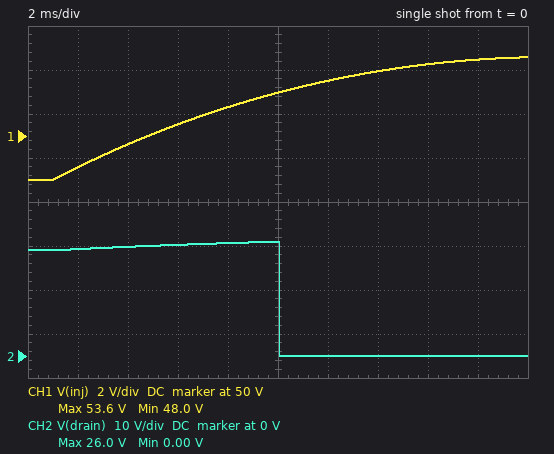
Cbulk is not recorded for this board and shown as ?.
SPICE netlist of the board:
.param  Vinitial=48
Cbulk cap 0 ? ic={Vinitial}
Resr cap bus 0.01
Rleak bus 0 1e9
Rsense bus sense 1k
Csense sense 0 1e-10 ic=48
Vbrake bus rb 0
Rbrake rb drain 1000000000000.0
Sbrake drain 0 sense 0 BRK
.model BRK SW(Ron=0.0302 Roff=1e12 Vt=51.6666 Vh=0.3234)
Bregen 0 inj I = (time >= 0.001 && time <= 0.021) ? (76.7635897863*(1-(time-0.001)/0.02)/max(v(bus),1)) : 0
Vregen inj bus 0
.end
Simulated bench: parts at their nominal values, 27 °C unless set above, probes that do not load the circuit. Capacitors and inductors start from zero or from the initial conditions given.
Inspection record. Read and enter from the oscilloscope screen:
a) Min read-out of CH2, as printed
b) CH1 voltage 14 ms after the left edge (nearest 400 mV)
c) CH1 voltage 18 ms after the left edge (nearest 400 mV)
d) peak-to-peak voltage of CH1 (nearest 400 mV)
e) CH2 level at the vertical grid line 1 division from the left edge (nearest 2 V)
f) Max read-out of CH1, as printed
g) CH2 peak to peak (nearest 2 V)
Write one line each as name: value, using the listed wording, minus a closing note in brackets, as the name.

Min read-out of CH2, as printed: 0.00 V
CH1 voltage 14 ms after the left edge: 52.8 V
CH1 voltage 18 ms after the left edge: 53.6 V
peak-to-peak voltage of CH1: 5.6 V
CH2 level at the vertical grid line 1 division from the left edge: 24 V
Max read-out of CH1, as printed: 53.6 V
CH2 peak to peak: 26 V
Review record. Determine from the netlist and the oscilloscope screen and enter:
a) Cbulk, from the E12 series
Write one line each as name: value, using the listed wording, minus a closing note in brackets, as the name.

Cbulk, from the E12 series: 2.7 mF
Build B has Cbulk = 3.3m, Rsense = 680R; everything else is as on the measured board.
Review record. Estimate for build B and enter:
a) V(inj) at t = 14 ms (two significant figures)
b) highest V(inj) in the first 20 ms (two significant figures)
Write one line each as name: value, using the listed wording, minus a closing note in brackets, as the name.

V(inj) at t = 14 ms: 52 V
highest V(inj) in the first 20 ms: 53 V
